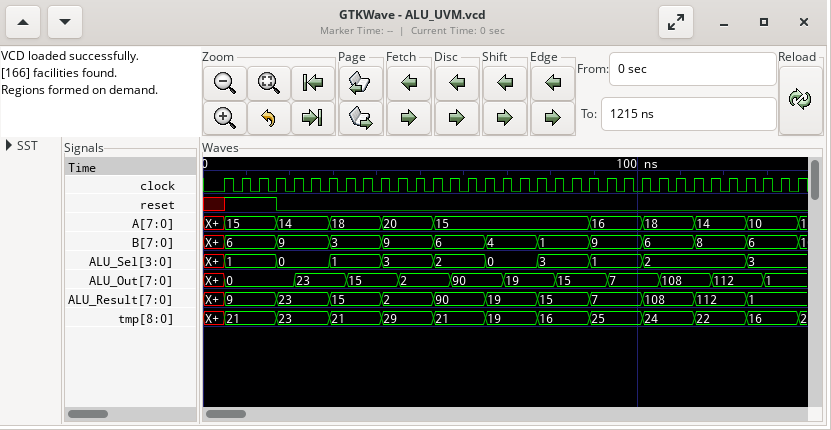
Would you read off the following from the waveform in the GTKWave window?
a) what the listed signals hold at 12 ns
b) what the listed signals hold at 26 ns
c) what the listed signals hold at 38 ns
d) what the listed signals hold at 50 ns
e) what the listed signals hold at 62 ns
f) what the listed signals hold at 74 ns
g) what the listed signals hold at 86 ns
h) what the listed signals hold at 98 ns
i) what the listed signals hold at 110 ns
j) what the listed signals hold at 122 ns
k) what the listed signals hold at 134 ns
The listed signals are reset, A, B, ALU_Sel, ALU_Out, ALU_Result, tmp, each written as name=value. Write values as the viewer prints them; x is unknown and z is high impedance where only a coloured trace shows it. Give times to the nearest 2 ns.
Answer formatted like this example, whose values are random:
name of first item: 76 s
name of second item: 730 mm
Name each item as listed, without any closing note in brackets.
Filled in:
what the listed signals hold at 12 ns: reset=1, A=15, B=6, ALU_Sel=1, ALU_Out=0, ALU_Result=9, tmp=21
what the listed signals hold at 26 ns: reset=0, A=14, B=9, ALU_Sel=0, ALU_Out=23, ALU_Result=23, tmp=23
what the listed signals hold at 38 ns: reset=0, A=18, B=3, ALU_Sel=1, ALU_Out=15, ALU_Result=15, tmp=21
what the listed signals hold at 50 ns: reset=0, A=20, B=9, ALU_Sel=3, ALU_Out=2, ALU_Result=2, tmp=29
what the listed signals hold at 62 ns: reset=0, A=15, B=6, ALU_Sel=2, ALU_Out=90, ALU_Result=90, tmp=21
what the listed signals hold at 74 ns: reset=0, A=15, B=4, ALU_Sel=0, ALU_Out=19, ALU_Result=19, tmp=19
what the listed signals hold at 86 ns: reset=0, A=15, B=1, ALU_Sel=3, ALU_Out=15, ALU_Result=15, tmp=16
what the listed signals hold at 98 ns: reset=0, A=16, B=9, ALU_Sel=1, ALU_Out=7, ALU_Result=7, tmp=25
what the listed signals hold at 110 ns: reset=0, A=18, B=6, ALU_Sel=2, ALU_Out=108, ALU_Result=108, tmp=24
what the listed signals hold at 122 ns: reset=0, A=14, B=8, ALU_Sel=2, ALU_Out=112, ALU_Result=112, tmp=22
what the listed signals hold at 134 ns: reset=0, A=10, B=6, ALU_Sel=3, ALU_Out=1, ALU_Result=1, tmp=16
